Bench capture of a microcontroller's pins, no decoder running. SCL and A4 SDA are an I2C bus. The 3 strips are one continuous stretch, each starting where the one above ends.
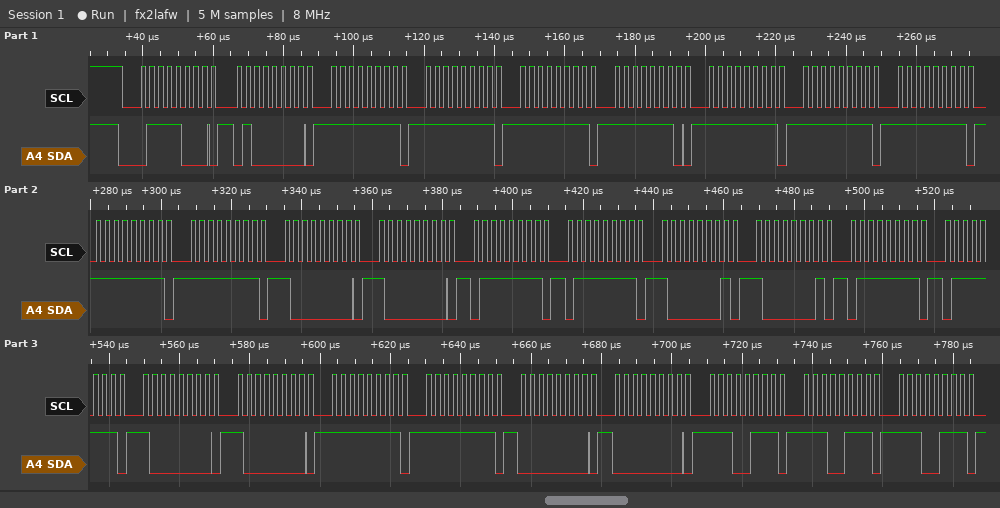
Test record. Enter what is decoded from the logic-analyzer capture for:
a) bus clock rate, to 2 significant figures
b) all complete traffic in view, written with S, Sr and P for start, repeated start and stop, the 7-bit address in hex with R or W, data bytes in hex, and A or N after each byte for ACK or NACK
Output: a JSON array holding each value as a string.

["400 kHz", "S 3CW A 40 A FF A FF A FF A FE A FF A FF A FF A FF A FF A 80 A 80 A 7F A 7F A 81 A 81 A 7F A 7F A 80 A 80 A FF A FF A 00 A 00 A E7 A E7 A E7 A"]
